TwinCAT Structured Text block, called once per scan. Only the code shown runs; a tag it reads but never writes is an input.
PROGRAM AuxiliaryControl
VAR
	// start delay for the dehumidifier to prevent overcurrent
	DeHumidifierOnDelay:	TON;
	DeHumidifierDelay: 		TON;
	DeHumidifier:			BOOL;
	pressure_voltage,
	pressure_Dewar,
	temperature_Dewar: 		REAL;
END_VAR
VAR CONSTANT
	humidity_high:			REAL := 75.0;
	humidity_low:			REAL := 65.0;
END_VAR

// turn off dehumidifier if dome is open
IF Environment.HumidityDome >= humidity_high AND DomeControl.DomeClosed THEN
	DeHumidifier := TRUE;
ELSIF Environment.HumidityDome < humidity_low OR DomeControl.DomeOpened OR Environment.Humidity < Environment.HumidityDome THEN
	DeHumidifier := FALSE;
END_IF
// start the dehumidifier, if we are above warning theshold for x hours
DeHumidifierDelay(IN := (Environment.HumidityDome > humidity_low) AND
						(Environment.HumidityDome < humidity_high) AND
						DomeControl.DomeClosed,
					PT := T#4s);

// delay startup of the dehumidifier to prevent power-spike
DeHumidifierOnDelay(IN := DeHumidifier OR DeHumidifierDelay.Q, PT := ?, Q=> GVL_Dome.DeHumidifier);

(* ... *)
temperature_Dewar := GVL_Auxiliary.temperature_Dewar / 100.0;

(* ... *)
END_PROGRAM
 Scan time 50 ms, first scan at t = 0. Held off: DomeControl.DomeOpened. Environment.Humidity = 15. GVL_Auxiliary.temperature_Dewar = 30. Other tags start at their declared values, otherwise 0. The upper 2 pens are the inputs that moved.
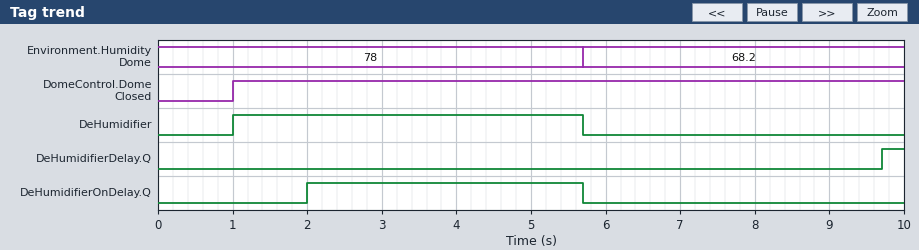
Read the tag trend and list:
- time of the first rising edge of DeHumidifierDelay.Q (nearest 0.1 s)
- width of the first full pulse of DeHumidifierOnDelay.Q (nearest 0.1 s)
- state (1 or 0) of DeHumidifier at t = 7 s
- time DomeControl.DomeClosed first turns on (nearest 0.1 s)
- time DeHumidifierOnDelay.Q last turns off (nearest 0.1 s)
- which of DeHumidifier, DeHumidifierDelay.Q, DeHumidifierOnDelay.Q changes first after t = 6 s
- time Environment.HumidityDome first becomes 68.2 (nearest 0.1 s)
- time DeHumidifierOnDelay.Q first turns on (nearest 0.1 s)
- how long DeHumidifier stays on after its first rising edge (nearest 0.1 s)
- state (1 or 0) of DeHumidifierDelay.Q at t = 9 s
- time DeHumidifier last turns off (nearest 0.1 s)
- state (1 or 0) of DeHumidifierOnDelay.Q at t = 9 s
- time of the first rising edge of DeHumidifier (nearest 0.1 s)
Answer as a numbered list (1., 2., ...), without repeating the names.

1. 9.7 s
2. 3.7 s
3. 0
4. 1.0 s
5. 5.7 s
6. DeHumidifierDelay.Q
7. 5.7 s
8. 2.0 s
9. 4.7 s
10. 0
11. 5.7 s
12. 0
13. 1.0 s
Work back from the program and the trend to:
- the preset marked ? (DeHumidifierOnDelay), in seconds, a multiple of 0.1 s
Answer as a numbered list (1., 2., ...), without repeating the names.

1. 1.0 s
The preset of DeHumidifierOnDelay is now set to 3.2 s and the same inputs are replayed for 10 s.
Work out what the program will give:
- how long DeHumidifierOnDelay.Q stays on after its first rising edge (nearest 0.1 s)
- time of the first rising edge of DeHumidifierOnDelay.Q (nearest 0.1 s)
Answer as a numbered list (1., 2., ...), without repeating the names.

1. 1.5 s
2. 4.2 s
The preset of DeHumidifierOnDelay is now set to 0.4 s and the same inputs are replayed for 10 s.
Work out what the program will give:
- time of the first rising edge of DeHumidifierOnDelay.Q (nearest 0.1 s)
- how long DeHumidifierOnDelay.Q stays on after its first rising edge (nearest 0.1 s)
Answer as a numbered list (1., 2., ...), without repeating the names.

1. 1.4 s
2. 4.3 s
